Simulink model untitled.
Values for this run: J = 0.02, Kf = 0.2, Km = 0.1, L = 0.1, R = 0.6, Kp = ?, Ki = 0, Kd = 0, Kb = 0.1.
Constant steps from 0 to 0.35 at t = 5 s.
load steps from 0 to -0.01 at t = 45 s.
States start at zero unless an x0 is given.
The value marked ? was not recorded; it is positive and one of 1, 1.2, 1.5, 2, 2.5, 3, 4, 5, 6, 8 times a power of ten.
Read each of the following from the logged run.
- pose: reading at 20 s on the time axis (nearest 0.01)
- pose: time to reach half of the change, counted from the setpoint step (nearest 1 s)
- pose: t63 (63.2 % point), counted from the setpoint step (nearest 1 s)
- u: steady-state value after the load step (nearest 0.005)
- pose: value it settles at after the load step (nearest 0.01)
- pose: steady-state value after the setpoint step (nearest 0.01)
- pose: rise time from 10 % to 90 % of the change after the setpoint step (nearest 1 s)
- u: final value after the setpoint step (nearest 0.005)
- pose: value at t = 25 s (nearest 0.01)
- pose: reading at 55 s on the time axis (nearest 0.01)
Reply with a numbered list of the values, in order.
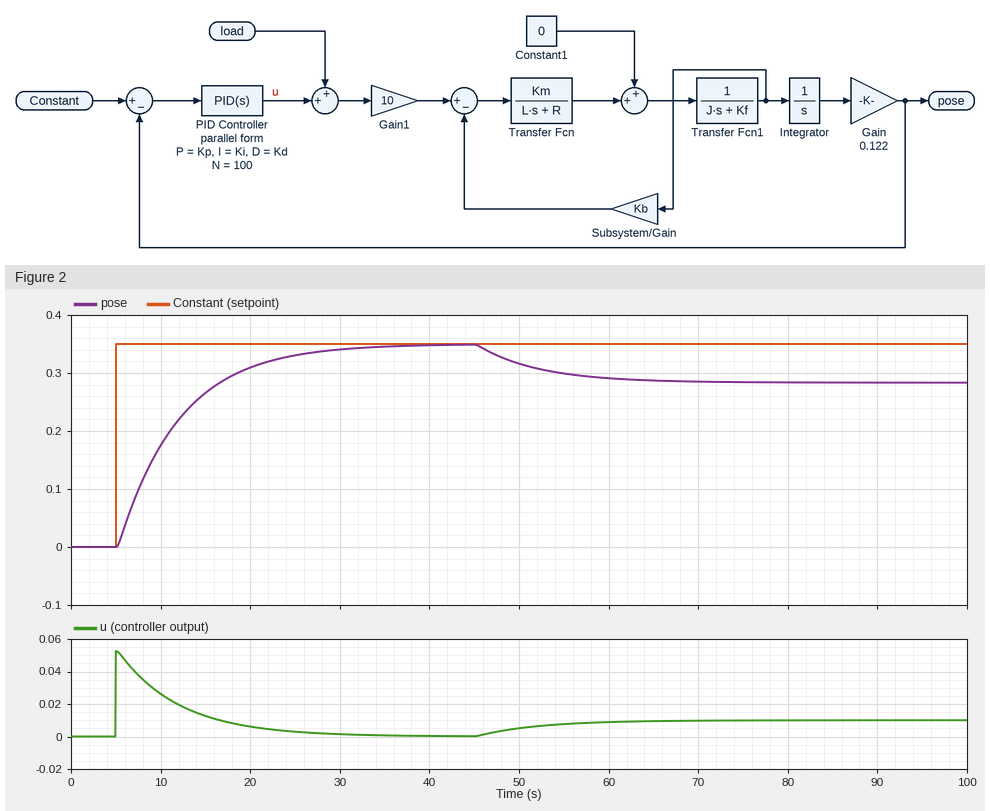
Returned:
1. 0.31
2. 5 s
3. 7 s
4. 0.010
5. 0.28
6. 0.35
7. 15 s
8. 0.000
9. 0.33
10. 0.30
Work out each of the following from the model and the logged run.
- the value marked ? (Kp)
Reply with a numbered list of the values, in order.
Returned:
1. 0.15
